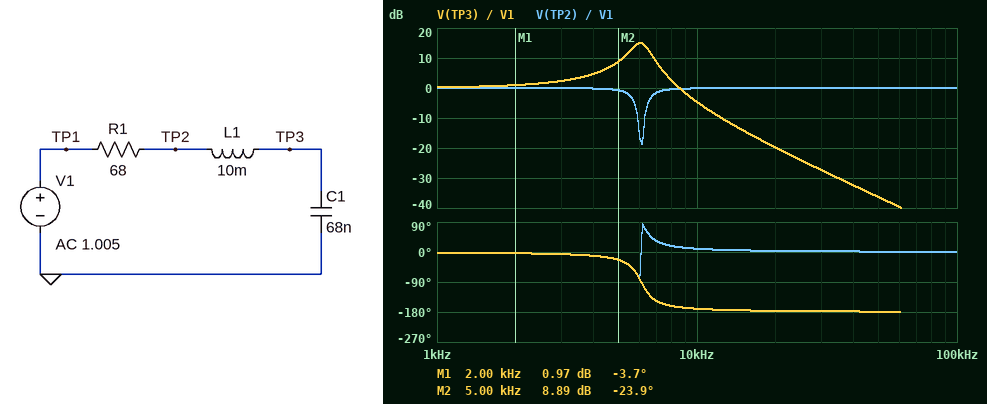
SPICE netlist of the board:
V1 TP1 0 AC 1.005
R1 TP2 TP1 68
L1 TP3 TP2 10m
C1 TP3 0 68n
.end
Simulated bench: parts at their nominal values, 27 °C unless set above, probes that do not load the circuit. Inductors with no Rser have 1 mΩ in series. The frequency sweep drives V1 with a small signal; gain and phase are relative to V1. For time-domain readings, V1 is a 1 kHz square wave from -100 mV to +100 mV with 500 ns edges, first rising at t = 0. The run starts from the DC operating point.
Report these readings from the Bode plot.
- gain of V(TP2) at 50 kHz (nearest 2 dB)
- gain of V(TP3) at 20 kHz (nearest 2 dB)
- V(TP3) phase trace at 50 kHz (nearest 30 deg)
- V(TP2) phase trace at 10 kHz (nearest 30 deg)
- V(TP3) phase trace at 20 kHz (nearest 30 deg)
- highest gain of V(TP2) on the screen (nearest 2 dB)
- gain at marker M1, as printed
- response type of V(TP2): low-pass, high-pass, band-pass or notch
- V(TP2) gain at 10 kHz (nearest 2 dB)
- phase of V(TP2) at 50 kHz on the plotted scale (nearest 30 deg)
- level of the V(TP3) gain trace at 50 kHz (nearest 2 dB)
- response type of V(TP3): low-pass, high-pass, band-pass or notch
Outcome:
0 dB
-20 dB
-180 deg
0 deg
-180 deg
0 dB
0.97 dB
notch
0 dB
0 deg
-36 dB
low-pass
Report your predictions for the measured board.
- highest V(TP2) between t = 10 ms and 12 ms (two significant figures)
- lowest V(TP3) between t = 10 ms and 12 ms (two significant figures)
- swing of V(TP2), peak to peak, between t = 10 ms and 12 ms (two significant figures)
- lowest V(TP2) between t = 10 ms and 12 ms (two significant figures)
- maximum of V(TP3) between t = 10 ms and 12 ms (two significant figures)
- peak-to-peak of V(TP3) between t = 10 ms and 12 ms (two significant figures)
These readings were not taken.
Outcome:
120 mV
-230 mV
240 mV
-120 mV
230 mV
460 mV
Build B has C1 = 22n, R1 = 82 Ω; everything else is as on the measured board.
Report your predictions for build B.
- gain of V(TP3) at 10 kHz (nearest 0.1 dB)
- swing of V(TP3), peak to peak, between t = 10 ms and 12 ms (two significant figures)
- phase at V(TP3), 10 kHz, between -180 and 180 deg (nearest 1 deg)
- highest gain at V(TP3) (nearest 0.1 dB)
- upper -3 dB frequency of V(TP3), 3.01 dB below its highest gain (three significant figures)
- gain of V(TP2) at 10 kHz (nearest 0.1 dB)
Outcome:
15.2 dB
550 mV
-41 deg
18.3 dB
11.3 kHz
-2.4 dB
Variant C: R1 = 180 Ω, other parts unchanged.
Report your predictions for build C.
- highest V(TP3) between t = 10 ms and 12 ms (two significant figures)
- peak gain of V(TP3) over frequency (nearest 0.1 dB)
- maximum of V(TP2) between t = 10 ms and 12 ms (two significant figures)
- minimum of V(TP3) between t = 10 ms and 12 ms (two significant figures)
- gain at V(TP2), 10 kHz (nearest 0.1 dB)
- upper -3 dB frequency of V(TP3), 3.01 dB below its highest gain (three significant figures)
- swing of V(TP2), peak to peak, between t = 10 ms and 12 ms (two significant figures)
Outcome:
190 mV
6.8 dB
130 mV
-190 mV
-0.8 dB
7.08 kHz
260 mV
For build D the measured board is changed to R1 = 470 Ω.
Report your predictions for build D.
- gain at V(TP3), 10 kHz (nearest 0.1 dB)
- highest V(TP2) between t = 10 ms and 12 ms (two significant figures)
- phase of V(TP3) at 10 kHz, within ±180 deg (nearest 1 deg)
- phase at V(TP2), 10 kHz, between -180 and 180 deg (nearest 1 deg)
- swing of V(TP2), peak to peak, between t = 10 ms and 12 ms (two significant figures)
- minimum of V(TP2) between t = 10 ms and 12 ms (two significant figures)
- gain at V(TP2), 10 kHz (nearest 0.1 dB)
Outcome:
-8.4 dB
110 mV
-130 deg
50 deg
220 mV
-110 mV
-3.8 dB
